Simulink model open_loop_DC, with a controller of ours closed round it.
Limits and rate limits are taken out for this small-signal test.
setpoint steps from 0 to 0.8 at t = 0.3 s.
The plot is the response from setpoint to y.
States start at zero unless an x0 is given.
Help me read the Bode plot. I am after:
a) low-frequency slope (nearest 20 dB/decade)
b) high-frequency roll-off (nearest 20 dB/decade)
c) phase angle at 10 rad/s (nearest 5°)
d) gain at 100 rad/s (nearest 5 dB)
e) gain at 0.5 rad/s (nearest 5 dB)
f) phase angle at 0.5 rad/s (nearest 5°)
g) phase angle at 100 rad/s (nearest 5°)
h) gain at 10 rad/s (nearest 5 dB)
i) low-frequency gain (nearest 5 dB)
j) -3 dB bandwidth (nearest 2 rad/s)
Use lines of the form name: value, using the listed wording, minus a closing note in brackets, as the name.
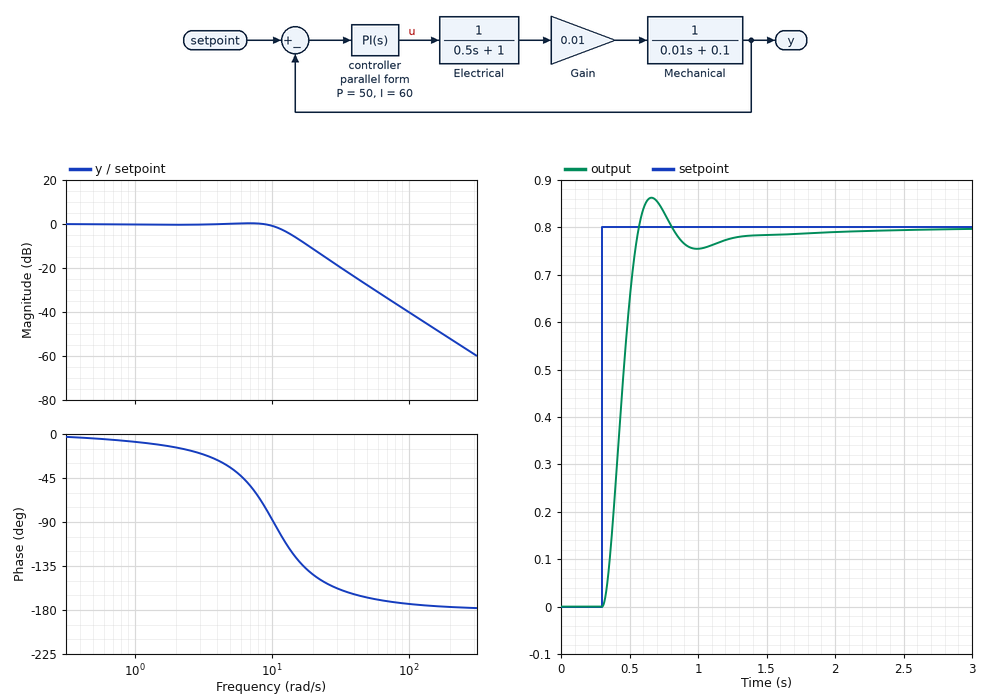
low-frequency slope: 0 dB/decade
high-frequency roll-off: -40 dB/decade
phase angle at 10 rad/s: -85°
gain at 100 rad/s: -40 dB
gain at 0.5 rad/s: 0 dB
phase angle at 0.5 rad/s: -5°
phase angle at 100 rad/s: -175°
gain at 10 rad/s: 0 dB
low-frequency gain: 0 dB
-3 dB bandwidth: 12 rad/s
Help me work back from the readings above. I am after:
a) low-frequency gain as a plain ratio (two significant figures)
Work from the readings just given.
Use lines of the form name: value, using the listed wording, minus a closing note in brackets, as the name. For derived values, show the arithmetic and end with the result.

low-frequency gain as a plain ratio: 10^(0 / 20) = 1.0
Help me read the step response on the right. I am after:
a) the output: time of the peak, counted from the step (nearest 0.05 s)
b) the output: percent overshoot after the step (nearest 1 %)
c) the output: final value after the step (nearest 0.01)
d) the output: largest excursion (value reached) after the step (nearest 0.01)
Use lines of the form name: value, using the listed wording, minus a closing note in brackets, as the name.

the output: time of the peak, counted from the step: 0.35 s
the output: percent overshoot after the step: 8 %
the output: final value after the step: 0.80
the output: largest excursion (value reached) after the step: 0.86
